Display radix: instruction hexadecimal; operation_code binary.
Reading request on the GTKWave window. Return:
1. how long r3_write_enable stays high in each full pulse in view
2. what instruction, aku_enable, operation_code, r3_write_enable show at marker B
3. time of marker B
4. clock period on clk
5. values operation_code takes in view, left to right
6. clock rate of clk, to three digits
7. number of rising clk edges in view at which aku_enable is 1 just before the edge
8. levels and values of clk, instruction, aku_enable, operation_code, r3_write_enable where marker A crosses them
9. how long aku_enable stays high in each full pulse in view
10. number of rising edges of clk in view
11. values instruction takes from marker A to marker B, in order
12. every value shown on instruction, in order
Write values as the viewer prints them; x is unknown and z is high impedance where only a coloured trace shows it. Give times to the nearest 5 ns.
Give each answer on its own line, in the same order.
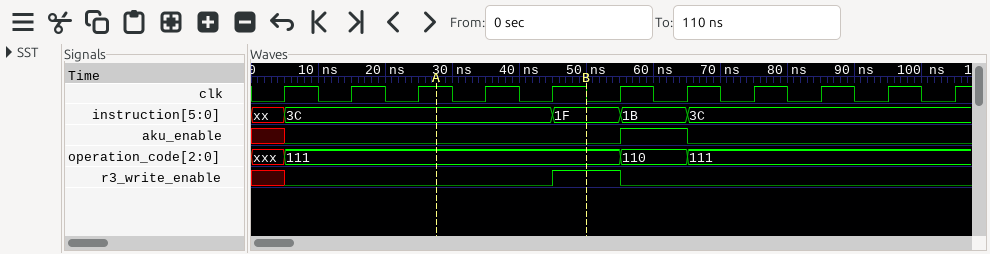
10 ns
instruction=1F, aku_enable=0, operation_code=111, r3_write_enable=1
50 ns
10 ns
xxx, 111, 110, 111
100 MHz
1
clk=1, instruction=3C, aku_enable=0, operation_code=111, r3_write_enable=0
10 ns
11
3C, 1F
xx, 3C, 1F, 1B, 3C
